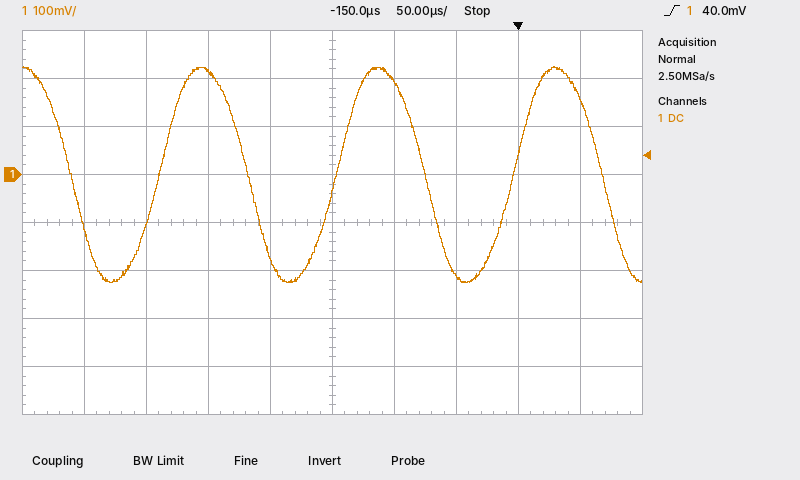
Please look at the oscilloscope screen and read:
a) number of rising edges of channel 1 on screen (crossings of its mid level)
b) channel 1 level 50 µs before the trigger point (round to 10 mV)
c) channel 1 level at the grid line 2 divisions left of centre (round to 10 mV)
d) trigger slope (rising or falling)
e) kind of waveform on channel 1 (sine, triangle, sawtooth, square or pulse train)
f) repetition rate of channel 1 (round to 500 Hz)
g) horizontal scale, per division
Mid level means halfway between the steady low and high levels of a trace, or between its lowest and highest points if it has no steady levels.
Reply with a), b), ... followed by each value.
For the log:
a) 3
b) -210 mV
c) 210 mV
d) rising
e) sine
f) 7.0 kHz
g) 50 µs
